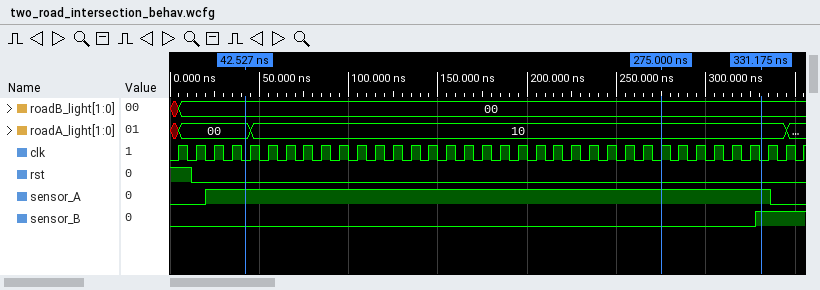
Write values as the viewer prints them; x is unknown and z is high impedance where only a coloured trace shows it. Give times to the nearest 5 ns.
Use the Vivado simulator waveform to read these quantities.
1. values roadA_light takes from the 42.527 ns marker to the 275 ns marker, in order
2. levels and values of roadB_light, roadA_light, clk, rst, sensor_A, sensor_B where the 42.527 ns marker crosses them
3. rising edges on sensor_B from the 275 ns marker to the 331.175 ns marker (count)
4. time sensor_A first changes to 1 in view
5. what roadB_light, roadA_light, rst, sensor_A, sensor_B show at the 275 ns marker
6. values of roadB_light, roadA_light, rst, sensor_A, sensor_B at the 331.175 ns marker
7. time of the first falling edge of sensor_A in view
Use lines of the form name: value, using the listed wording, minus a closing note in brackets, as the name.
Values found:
values roadA_light takes from the 42.527 ns marker to the 275 ns marker, in order: 00, 10
levels and values of roadB_light, roadA_light, clk, rst, sensor_A, sensor_B where the 42.527 ns marker crosses them: roadB_light=00, roadA_light=00, clk=0, rst=0, sensor_A=1, sensor_B=0
rising edges on sensor_B from the 275 ns marker to the 331.175 ns marker: 1
time sensor_A first changes to 1 in view: 20 ns
what roadB_light, roadA_light, rst, sensor_A, sensor_B show at the 275 ns marker: roadB_light=00, roadA_light=10, rst=0, sensor_A=1, sensor_B=0
values of roadB_light, roadA_light, rst, sensor_A, sensor_B at the 331.175 ns marker: roadB_light=00, roadA_light=10, rst=0, sensor_A=1, sensor_B=1
time of the first falling edge of sensor_A in view: 335 ns
